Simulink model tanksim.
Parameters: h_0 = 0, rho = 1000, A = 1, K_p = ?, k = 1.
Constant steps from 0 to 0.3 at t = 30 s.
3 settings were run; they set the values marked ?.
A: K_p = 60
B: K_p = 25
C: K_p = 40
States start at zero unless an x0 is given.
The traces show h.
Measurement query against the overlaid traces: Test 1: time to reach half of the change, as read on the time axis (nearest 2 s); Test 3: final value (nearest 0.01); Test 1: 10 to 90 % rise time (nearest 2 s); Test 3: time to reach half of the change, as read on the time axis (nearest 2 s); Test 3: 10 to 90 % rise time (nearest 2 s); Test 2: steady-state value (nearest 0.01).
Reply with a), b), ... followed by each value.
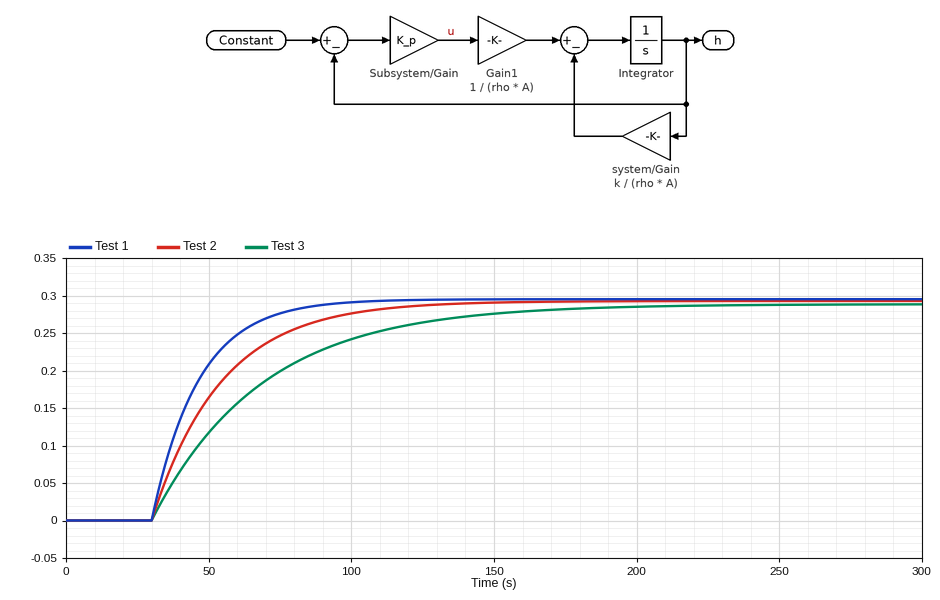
a) 42 s
b) 0.29
c) 36 s
d) 56 s
e) 84 s
f) 0.29
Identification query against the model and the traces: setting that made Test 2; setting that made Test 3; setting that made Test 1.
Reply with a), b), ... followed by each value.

a) C
b) B
c) A
